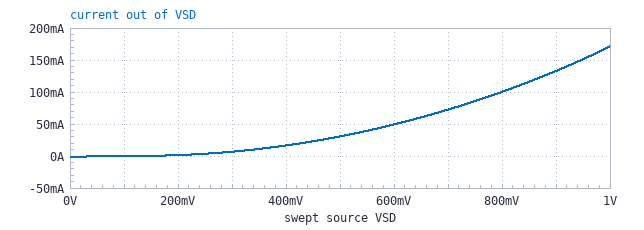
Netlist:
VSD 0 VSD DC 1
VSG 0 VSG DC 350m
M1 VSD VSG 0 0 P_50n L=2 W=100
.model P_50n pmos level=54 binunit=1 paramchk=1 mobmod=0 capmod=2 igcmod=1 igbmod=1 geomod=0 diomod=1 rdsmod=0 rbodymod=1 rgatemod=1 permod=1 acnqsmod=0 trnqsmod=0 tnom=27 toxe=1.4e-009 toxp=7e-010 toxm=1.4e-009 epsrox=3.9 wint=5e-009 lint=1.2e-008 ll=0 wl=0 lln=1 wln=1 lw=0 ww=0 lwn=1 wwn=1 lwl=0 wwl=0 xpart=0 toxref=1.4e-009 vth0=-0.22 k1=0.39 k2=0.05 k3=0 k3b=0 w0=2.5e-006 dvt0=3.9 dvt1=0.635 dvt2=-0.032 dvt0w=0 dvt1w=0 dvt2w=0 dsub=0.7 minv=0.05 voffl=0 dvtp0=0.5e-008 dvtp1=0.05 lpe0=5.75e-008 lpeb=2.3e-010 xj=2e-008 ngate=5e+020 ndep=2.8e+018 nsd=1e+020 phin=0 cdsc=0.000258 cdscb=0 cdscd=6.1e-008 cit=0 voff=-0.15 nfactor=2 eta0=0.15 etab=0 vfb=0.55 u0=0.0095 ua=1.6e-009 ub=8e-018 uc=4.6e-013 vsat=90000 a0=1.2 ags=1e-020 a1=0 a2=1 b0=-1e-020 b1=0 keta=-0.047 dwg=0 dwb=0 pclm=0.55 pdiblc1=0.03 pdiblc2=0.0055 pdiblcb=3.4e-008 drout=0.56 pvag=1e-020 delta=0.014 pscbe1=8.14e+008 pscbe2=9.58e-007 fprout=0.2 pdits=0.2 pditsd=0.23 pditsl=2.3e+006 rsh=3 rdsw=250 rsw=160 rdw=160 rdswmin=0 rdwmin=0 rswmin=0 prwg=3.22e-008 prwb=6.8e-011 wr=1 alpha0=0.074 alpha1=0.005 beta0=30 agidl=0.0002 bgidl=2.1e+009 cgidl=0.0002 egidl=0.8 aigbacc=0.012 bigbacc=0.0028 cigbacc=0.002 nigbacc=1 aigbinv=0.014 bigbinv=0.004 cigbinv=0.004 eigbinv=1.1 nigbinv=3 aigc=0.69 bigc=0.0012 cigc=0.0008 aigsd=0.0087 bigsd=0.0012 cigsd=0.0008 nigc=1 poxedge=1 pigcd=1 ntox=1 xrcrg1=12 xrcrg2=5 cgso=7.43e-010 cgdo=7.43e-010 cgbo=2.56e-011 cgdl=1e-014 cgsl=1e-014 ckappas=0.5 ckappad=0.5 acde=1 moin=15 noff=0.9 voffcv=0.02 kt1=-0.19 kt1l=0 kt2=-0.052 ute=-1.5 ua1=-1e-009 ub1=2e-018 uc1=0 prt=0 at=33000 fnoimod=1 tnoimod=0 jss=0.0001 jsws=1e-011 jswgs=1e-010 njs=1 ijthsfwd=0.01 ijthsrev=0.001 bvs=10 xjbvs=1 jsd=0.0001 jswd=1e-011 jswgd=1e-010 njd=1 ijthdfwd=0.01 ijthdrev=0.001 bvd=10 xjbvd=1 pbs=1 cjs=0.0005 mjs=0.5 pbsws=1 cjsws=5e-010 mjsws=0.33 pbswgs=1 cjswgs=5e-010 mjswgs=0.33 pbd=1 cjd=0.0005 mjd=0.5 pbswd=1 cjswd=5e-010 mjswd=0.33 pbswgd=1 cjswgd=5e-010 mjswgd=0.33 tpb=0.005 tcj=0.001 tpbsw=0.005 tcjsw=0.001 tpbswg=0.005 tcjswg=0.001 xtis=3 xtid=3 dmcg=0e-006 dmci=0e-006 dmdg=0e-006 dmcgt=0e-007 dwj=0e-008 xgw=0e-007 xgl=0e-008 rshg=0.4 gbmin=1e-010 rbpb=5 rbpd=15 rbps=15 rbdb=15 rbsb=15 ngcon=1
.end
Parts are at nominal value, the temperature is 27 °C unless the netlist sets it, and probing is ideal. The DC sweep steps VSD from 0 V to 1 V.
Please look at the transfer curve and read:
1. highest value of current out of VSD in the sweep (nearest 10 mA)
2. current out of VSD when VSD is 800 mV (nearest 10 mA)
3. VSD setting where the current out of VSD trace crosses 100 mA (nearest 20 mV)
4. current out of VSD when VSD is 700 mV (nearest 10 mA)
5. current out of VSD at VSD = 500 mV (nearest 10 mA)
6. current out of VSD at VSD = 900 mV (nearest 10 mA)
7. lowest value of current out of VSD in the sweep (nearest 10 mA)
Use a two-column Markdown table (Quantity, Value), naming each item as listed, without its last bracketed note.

| Quantity | Value |
|---|---|
| highest value of current out of VSD in the sweep | 170 mA |
| current out of VSD when VSD is 800 mV | 100 mA |
| VSD setting where the current out of VSD trace crosses 100 mA | 800 mV |
| current out of VSD when VSD is 700 mV | 70 mA |
| current out of VSD at VSD = 500 mV | 30 mA |
| current out of VSD at VSD = 900 mV | 130 mA |
| lowest value of current out of VSD in the sweep | 0 A |
